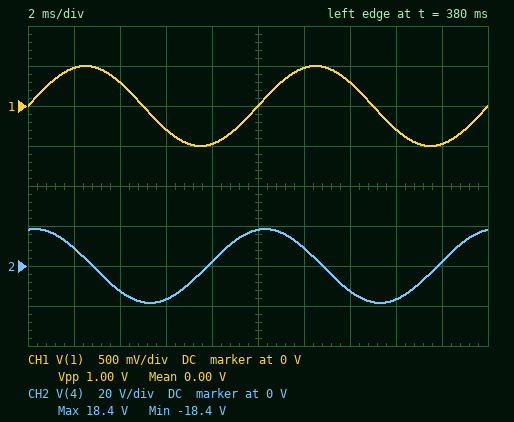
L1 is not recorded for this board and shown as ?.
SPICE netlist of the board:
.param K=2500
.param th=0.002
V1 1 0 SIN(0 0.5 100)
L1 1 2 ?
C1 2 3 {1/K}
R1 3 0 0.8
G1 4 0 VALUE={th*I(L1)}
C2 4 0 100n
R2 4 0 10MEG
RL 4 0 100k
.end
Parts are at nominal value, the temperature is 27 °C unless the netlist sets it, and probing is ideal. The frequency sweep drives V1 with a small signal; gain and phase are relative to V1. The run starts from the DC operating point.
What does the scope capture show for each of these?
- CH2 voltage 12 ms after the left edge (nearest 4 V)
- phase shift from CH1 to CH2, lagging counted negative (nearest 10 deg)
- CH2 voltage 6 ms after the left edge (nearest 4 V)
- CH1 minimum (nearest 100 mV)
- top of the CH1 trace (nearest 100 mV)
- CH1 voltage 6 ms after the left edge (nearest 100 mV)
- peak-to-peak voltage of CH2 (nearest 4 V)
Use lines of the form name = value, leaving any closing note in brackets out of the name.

CH2 voltage 12 ms after the left edge = 8 V
phase shift from CH1 to CH2, lagging counted negative = 80 deg
CH2 voltage 6 ms after the left edge = -16 V
CH1 minimum = -500 mV
top of the CH1 trace = 500 mV
CH1 voltage 6 ms after the left edge = -300 mV
peak-to-peak voltage of CH2 = 36 V
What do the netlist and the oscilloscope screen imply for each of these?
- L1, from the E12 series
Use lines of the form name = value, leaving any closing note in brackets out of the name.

L1, from the E12 series = 6.8 mH
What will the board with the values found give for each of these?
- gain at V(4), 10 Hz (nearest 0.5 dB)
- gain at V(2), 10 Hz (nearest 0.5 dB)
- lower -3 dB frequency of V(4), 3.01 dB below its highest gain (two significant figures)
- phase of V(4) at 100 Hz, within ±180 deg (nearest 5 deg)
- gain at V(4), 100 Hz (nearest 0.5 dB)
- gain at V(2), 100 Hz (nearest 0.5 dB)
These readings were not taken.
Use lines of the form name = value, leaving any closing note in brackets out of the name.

gain at V(4), 10 Hz = 12.5 dB
gain at V(2), 10 Hz = 0 dB
lower -3 dB frequency of V(4), 3.01 dB below its highest gain = 86 Hz
phase of V(4) at 100 Hz, within ±180 deg = 80 deg
gain at V(4), 100 Hz = 31.5 dB
gain at V(2), 100 Hz = 13.5 dB
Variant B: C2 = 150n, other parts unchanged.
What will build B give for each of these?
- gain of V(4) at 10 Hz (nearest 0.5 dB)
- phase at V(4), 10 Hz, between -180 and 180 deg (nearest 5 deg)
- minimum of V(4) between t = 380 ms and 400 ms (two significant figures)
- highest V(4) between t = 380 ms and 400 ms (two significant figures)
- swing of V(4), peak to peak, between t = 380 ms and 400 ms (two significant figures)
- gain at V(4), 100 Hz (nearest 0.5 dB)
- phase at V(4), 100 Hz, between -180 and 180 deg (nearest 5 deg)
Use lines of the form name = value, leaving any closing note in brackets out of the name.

gain of V(4) at 10 Hz = 11.5 dB
phase at V(4), 10 Hz, between -180 and 180 deg = -135 deg
minimum of V(4) between t = 380 ms and 400 ms = -12 V
highest V(4) between t = 380 ms and 400 ms = 12 V
swing of V(4), peak to peak, between t = 380 ms and 400 ms = 25 V
gain at V(4), 100 Hz = 28.0 dB
phase at V(4), 100 Hz, between -180 and 180 deg = 75 deg
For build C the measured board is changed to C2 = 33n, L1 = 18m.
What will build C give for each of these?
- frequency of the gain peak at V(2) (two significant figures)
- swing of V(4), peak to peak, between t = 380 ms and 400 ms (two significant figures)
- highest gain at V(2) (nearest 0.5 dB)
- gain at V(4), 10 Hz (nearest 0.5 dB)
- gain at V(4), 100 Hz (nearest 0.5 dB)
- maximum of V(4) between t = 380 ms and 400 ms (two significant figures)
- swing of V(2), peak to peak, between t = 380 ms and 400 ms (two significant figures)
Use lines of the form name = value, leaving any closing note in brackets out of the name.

frequency of the gain peak at V(2) = 59 Hz
swing of V(4), peak to peak, between t = 380 ms and 400 ms = 12 V
highest gain at V(2) = 18.5 dB
gain at V(4), 10 Hz = 14.0 dB
gain at V(4), 100 Hz = 21.5 dB
maximum of V(4) between t = 380 ms and 400 ms = 5.9 V
swing of V(2), peak to peak, between t = 380 ms and 400 ms = 550 mV
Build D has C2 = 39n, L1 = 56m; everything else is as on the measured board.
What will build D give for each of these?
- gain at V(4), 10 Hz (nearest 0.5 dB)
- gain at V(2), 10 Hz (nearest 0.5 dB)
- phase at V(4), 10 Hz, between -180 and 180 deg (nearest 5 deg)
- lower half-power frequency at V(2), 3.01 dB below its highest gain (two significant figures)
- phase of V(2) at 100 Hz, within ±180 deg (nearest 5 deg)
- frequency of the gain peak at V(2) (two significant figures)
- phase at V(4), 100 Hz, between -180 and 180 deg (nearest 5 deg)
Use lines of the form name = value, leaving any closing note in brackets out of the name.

gain at V(4), 10 Hz = 14.5 dB
gain at V(2), 10 Hz = 1.0 dB
phase at V(4), 10 Hz, between -180 and 180 deg = -105 deg
lower half-power frequency at V(2), 3.01 dB below its highest gain = 32 Hz
phase of V(2) at 100 Hz, within ±180 deg = -165 deg
frequency of the gain peak at V(2) = 34 Hz
phase at V(4), 100 Hz, between -180 and 180 deg = 25 deg
